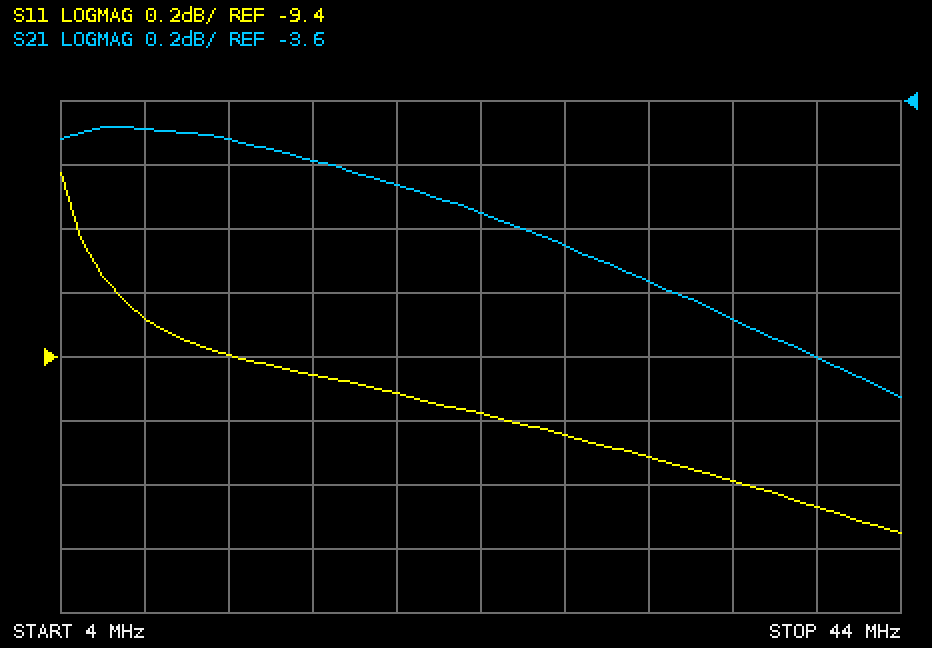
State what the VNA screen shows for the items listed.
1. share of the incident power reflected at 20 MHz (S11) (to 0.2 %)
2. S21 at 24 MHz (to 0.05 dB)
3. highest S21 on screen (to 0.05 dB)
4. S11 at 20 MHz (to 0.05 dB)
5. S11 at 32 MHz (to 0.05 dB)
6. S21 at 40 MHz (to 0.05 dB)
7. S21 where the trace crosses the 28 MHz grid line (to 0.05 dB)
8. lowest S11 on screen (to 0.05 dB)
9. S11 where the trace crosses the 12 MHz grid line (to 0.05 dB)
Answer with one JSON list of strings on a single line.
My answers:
["11.2 %", "-3.95 dB", "-3.70 dB", "-9.50 dB", "-9.70 dB", "-4.40 dB", "-4.05 dB", "-9.95 dB", "-9.40 dB"]
